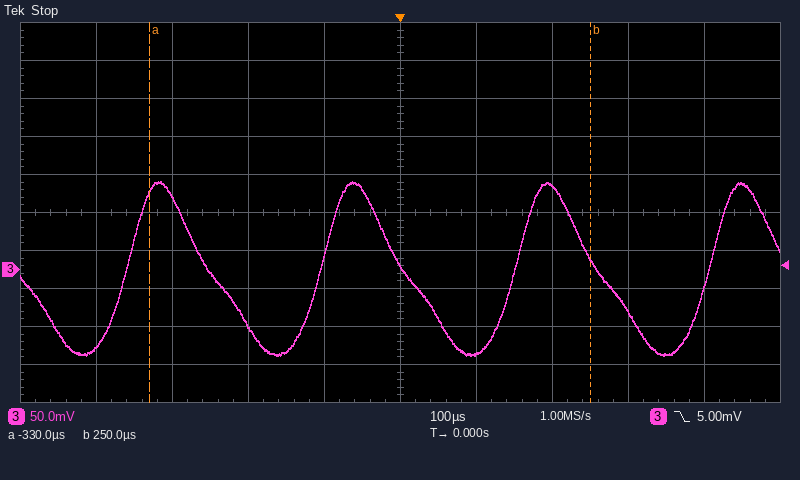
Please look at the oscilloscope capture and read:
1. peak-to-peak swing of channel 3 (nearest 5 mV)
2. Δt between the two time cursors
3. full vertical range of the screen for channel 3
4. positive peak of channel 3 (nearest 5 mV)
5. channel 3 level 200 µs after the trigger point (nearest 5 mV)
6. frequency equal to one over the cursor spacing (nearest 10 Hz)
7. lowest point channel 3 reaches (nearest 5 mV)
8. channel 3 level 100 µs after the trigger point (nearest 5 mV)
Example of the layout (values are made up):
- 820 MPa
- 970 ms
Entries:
- 230 mV
- 580 µs
- 500 mV
- 115 mV
- 110 mV
- 1.72 kHz
- -115 mV
- -110 mV
